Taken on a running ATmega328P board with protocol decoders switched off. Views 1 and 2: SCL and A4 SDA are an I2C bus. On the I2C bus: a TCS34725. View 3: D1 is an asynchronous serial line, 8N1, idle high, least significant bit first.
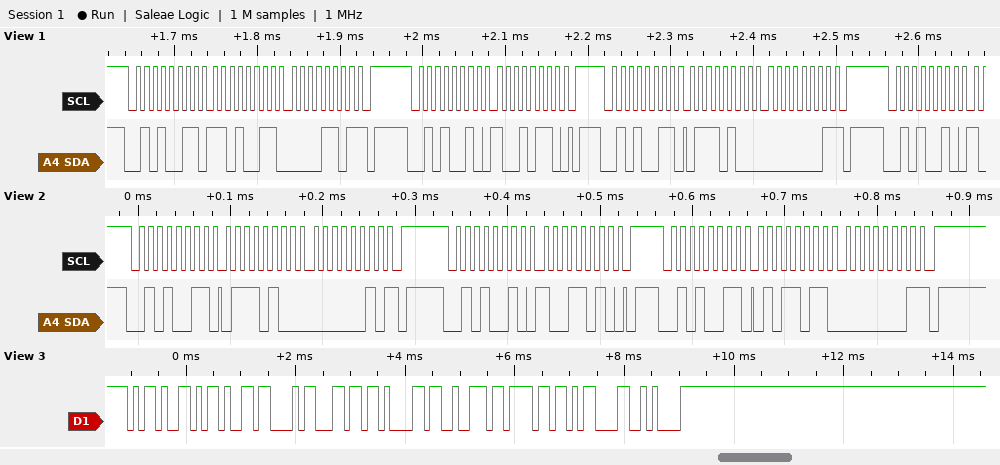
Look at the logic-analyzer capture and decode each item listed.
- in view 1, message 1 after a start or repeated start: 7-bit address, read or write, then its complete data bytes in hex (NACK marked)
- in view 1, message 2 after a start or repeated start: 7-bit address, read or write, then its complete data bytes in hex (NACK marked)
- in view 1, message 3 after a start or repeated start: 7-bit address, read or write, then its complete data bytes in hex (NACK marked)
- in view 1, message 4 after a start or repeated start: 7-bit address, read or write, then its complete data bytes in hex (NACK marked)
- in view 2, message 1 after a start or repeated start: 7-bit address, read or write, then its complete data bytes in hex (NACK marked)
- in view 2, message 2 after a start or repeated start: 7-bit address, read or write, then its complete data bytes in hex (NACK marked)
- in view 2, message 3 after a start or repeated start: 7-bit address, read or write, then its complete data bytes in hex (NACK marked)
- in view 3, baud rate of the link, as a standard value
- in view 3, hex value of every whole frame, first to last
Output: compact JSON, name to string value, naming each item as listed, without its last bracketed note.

{"in view 1, message 1 after a start or repeated start: 7-bit address, read or write, then its complete data bytes in hex": "0x29 read: D3 0D NACK", "in view 1, message 2 after a start or repeated start: 7-bit address, read or write, then its complete data bytes in hex": "0x29 write: 96", "in view 1, message 3 after a start or repeated start: 7-bit address, read or write, then its complete data bytes in hex": "0x29 read: 74 01 NACK", "in view 1, message 4 after a start or repeated start: 7-bit address, read or write, then its complete data bytes in hex": "0x29 write", "in view 2, message 1 after a start or repeated start: 7-bit address, read or write, then its complete data bytes in hex": "0x29 read: 74 02 NACK", "in view 2, message 2 after a start or repeated start: 7-bit address, read or write, then its complete data bytes in hex": "0x29 write: 9A", "in view 2, message 3 after a start or repeated start: 7-bit address, read or write, then its complete data bytes in hex": "0x29 read: 5B 01 NACK", "in view 3, baud rate of the link, as a standard value": "9600 baud", "in view 3, hex value of every whole frame, first to last": "0x2D 0x2D 0x43 0x6C 0x61 0x72 0x6F 0x0D 0x0A"}
